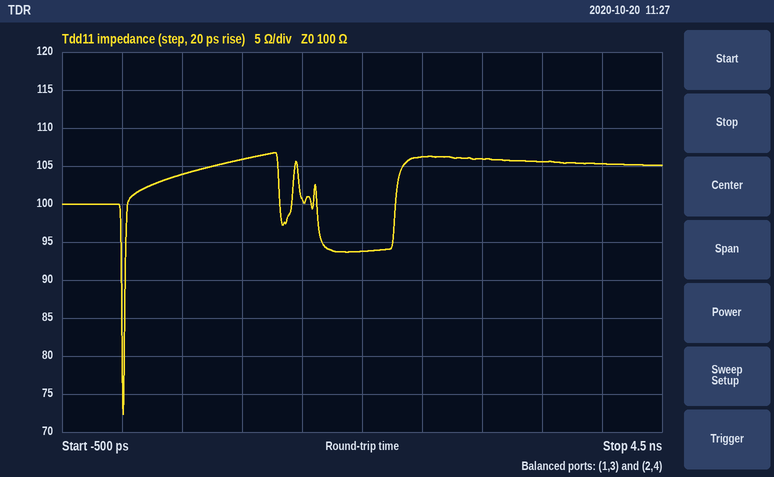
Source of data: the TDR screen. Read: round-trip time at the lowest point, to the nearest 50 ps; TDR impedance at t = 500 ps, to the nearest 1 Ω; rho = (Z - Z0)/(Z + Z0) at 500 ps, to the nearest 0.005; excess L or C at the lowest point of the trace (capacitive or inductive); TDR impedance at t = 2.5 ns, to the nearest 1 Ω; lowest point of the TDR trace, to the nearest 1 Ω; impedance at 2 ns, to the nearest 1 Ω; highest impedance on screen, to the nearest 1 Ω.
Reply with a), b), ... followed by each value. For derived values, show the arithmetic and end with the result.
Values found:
a) 0 ps
b) 104 Ω
c) (104 − 100)/(104 + 100) ≈ +0.020
d) capacitive
e) 106 Ω
f) 72 Ω
g) 94 Ω
h) 107 Ω
